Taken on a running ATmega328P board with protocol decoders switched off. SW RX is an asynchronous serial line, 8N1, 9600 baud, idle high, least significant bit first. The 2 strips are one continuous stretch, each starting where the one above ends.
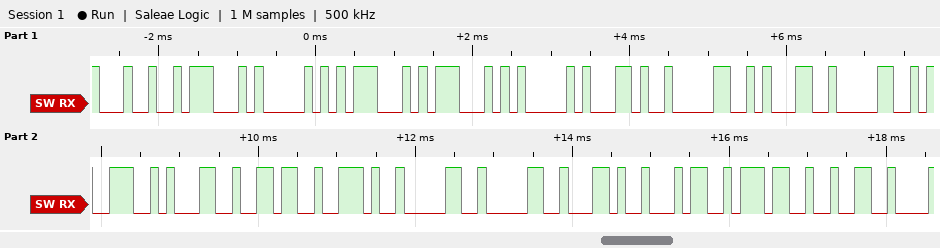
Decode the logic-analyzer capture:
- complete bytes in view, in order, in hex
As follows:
0x24 0x47 0x50 0x47 0x47 0x41 0x2C 0x30 0x31 0x30 0x39 0x31 0x36 0x2E 0x30 0x30 0x2C 0x34 0x37 0x32
